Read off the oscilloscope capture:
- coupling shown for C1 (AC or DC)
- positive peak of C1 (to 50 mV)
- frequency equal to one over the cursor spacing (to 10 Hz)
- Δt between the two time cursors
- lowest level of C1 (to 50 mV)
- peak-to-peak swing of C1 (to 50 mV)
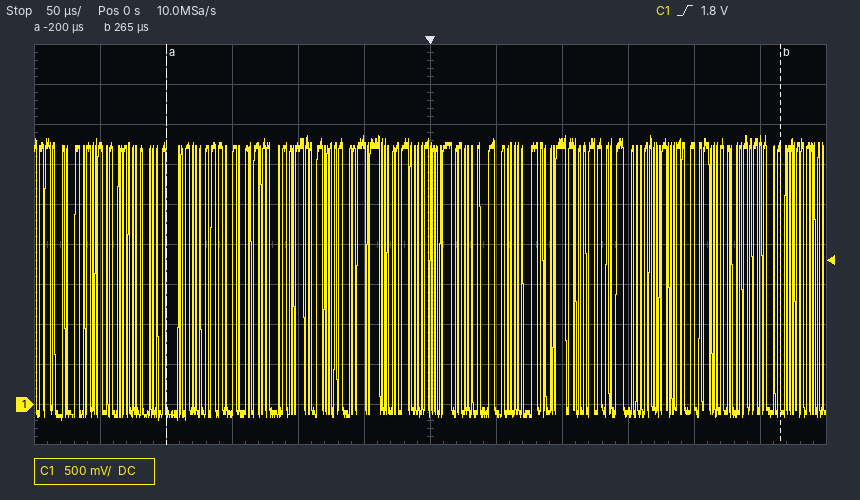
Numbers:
DC
3.35 V
2.15 kHz
465 µs
-200 mV
3.55 V
